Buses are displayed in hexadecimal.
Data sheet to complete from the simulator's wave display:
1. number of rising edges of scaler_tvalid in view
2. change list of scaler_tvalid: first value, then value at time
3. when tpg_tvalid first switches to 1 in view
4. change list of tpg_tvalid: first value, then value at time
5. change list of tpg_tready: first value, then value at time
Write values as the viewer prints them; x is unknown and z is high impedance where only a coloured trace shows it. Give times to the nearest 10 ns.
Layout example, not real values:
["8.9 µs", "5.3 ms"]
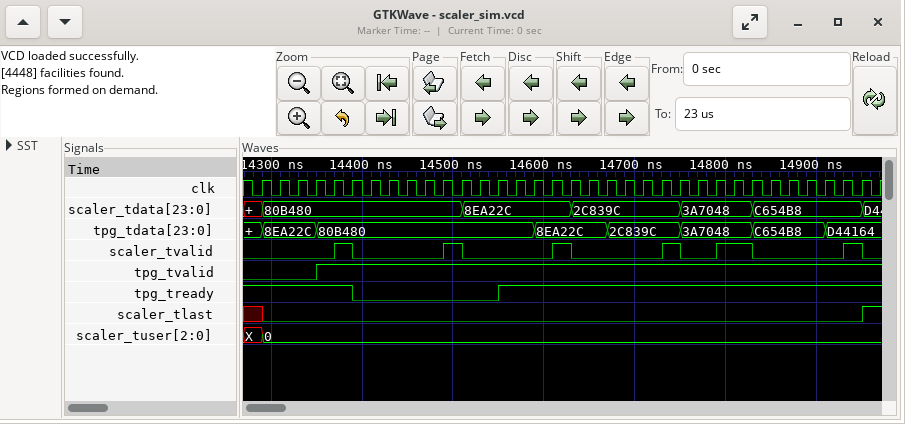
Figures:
["6", "0, 1 at 14370 ns, 0 at 14390 ns, 1 at 14490 ns, 0 at 14510 ns, 1 at 14610 ns, 0 at 14630 ns, 1 at 14730 ns, 0 at 14750 ns, 1 at 14790 ns, 0 at 14830 ns, 1 at 14930 ns, 0 at 14950 ns", "14350 ns", "0, 1 at 14350 ns", "1, 0 at 14390 ns, 1 at 14550 ns"]
